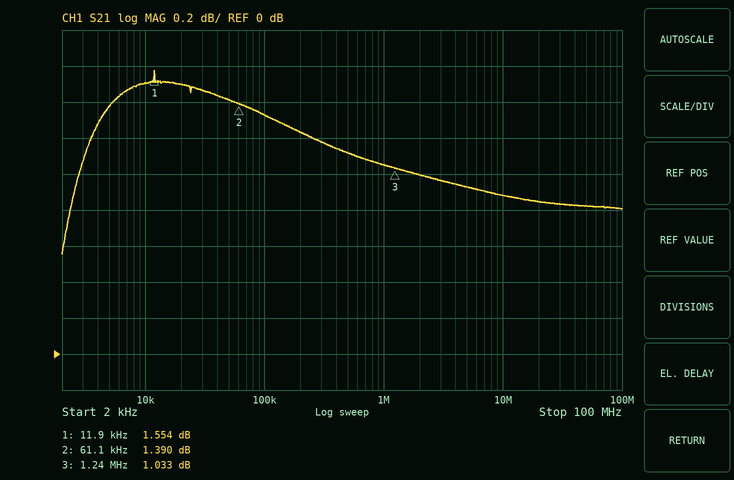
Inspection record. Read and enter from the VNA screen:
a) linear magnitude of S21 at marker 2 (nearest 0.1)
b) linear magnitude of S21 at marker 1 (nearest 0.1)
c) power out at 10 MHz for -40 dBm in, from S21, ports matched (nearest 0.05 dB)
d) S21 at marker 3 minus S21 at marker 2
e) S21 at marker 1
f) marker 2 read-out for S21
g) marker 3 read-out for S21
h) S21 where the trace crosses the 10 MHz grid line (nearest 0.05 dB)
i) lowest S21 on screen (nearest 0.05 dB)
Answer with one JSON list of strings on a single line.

["1.2", "1.2", "-39.10 dBm", "-0.357 dB", "1.554 dB", "1.390 dB", "1.033 dB", "0.90 dB", "0.55 dB"]
